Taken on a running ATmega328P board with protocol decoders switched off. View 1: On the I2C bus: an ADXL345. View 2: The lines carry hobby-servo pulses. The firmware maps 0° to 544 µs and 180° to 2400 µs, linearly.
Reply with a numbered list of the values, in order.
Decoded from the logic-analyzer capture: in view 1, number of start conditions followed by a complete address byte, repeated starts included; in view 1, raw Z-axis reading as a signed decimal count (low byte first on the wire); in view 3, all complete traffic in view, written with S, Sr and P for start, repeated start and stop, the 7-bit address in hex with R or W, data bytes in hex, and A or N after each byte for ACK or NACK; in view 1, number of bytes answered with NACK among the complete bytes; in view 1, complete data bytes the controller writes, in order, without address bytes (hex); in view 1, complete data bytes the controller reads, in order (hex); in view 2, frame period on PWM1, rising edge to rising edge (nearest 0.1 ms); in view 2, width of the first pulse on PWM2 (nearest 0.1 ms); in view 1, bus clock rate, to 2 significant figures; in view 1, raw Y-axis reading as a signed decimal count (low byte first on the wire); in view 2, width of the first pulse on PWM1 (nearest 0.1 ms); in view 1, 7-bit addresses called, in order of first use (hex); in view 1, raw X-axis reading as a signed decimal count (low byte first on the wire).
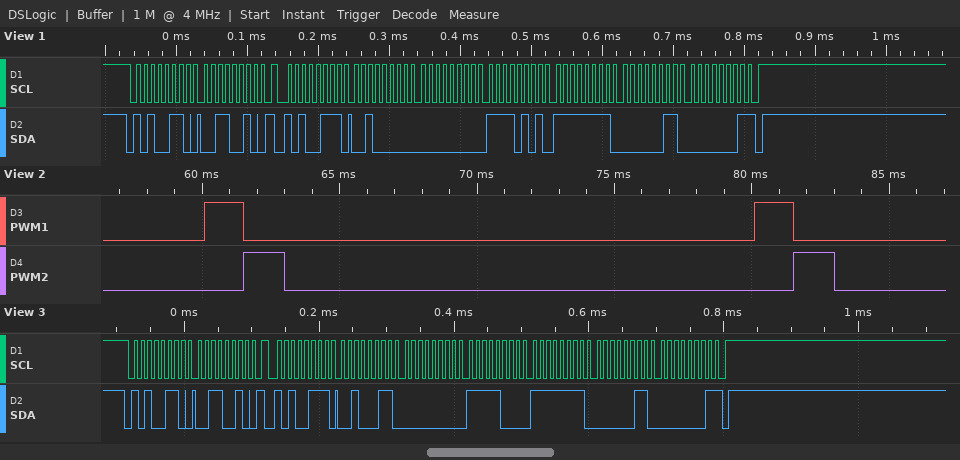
1. 2
2. 259
3. S 53W A 32 A Sr 53R A 23 A 00 A F8 A FF A 03 A 01 N P
4. 1
5. 32
6. 20 00 F5 FF 03 01
7. 20.0 ms
8. 1.5 ms
9. 100 kHz
10. -11
11. 1.4 ms
12. 0x53
13. 32
